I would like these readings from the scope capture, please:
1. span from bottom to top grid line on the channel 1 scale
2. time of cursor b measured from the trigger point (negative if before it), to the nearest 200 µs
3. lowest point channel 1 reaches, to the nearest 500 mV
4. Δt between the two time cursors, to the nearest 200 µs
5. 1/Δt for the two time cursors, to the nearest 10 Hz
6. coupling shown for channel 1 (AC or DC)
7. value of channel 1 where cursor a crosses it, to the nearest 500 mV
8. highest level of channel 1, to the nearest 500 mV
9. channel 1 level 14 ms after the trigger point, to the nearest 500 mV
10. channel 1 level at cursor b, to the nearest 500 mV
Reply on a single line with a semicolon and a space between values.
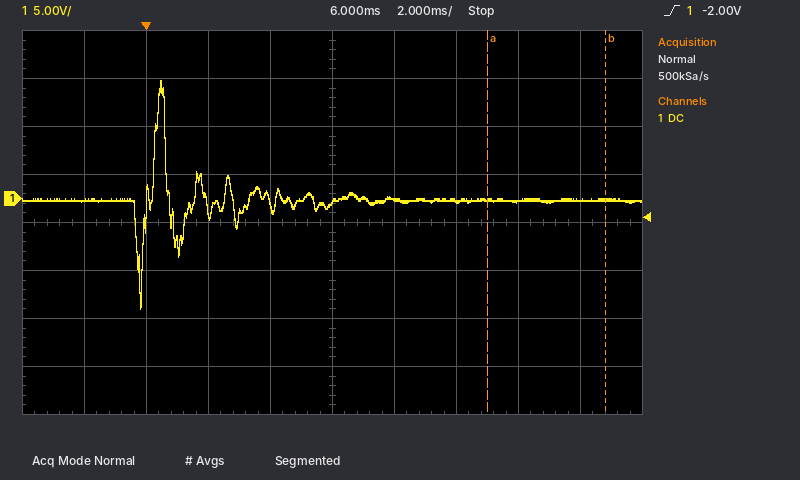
40 V; +14.8 ms; -11.5 V; 3.8 ms; 260 Hz; DC; 0.0 V; 12.5 V; 0.0 V; 0.0 V
